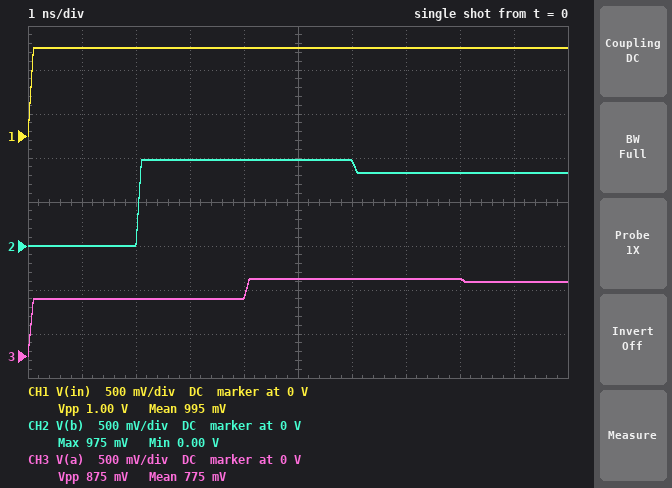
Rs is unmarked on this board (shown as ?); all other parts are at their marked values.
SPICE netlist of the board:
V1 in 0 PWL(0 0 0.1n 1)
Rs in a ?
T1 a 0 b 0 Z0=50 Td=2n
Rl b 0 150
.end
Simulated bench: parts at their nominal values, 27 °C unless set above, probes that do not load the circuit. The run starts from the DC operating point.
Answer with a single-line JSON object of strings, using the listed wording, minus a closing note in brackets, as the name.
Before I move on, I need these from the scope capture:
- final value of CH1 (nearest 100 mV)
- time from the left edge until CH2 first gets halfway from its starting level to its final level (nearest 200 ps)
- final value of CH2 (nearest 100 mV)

{"final value of CH1": "1.0 V", "time from the left edge until CH2 first gets halfway from its starting level to its final level": "2.0 ns", "final value of CH2": "800 mV"}
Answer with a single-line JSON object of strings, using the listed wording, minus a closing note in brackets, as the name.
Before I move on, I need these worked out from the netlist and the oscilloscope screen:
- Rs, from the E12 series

{"Rs, from the E12 series": "27 Ω"}
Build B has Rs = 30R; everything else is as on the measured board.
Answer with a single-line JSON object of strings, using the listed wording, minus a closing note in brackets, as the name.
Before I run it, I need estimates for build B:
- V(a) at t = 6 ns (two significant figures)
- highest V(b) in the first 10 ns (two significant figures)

{"V(a) at t = 6 ns": "860 mV", "highest V(b) in the first 10 ns": "940 mV"}
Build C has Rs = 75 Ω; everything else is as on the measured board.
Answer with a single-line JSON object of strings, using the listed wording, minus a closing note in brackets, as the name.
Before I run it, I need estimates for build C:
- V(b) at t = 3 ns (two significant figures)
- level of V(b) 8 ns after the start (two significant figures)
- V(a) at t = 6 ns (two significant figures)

{"V(b) at t = 3 ns": "600 mV", "level of V(b) 8 ns after the start": "660 mV", "V(a) at t = 6 ns": "640 mV"}
